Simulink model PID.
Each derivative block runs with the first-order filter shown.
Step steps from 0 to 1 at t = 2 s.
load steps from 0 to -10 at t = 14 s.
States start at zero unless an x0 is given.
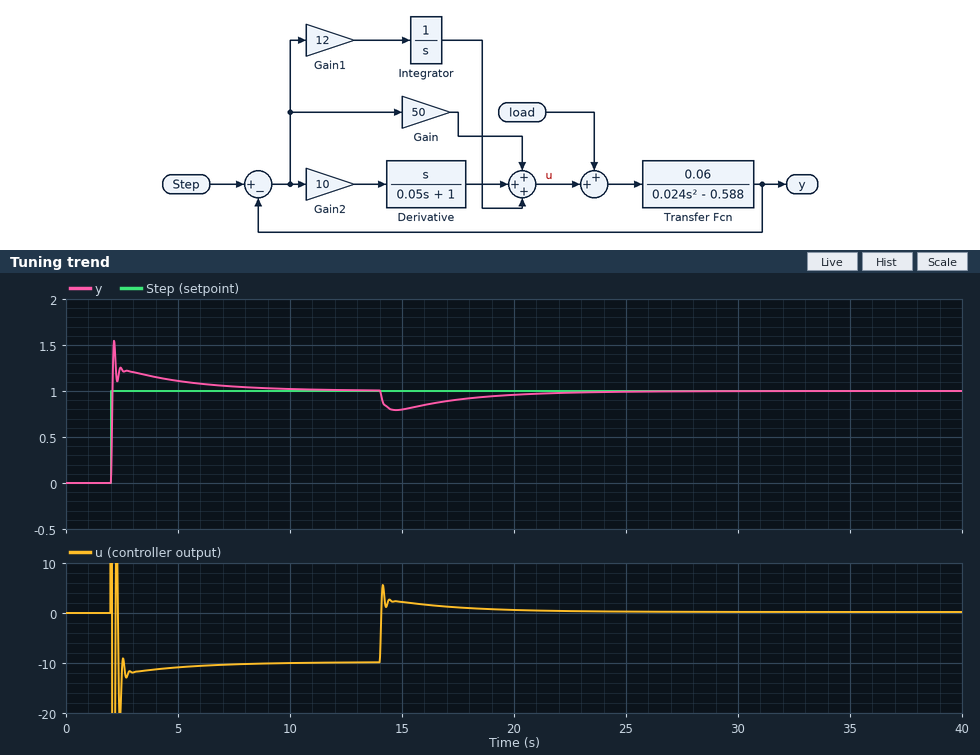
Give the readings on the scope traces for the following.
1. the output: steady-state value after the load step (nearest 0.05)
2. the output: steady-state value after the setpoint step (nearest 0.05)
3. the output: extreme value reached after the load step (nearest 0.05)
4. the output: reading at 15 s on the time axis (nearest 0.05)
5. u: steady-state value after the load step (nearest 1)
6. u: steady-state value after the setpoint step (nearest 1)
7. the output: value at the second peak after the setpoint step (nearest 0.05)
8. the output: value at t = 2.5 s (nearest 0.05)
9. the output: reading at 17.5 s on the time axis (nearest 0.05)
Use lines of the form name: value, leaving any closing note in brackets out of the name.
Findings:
the output: steady-state value after the load step: 1.00
the output: steady-state value after the setpoint step: 1.00
the output: extreme value reached after the load step: 0.80
the output: reading at 15 s on the time axis: 0.80
u: steady-state value after the load step: 0
u: steady-state value after the setpoint step: -10
the output: value at the second peak after the setpoint step: 1.25
the output: value at t = 2.5 s: 1.25
the output: reading at 17.5 s on the time axis: 0.90
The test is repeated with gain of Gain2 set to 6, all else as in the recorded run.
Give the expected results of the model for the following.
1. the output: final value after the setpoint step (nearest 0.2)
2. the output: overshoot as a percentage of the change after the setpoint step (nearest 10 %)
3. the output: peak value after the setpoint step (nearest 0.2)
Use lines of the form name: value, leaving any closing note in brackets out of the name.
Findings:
the output: final value after the setpoint step: 1.0
the output: overshoot as a percentage of the change after the setpoint step: 70 %
the output: peak value after the setpoint step: 1.6
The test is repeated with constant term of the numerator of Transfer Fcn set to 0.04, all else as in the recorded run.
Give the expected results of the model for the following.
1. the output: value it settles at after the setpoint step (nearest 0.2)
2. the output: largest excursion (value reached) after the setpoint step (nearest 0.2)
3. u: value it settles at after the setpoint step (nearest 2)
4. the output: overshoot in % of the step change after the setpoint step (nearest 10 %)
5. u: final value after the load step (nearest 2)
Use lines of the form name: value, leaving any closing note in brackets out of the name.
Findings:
the output: value it settles at after the setpoint step: 1.0
the output: largest excursion (value reached) after the setpoint step: 1.6
u: value it settles at after the setpoint step: -14
the output: overshoot in % of the step change after the setpoint step: 60 %
u: final value after the load step: -4
